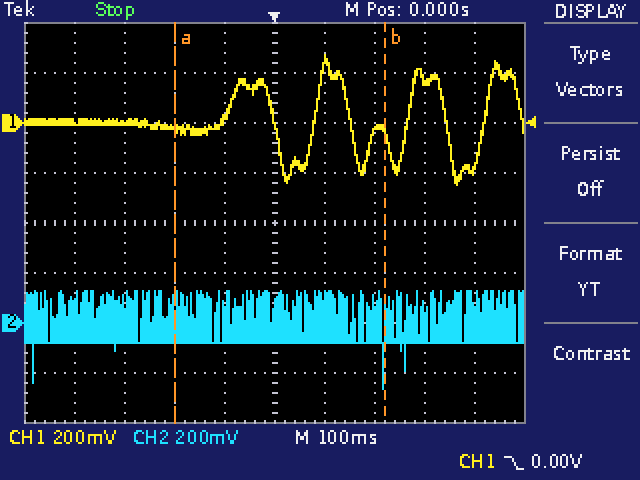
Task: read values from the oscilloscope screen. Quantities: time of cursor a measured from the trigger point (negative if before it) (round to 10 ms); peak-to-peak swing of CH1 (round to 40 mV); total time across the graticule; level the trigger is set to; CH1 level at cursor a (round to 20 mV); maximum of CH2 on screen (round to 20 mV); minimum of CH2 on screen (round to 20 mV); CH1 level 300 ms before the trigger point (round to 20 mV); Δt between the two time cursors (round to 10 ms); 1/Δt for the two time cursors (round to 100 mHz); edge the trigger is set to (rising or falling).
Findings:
-200 ms
520 mV
1 s
0.00 V
-20 mV
120 mV
-260 mV
0 mV
420 ms
2.4 Hz
falling
